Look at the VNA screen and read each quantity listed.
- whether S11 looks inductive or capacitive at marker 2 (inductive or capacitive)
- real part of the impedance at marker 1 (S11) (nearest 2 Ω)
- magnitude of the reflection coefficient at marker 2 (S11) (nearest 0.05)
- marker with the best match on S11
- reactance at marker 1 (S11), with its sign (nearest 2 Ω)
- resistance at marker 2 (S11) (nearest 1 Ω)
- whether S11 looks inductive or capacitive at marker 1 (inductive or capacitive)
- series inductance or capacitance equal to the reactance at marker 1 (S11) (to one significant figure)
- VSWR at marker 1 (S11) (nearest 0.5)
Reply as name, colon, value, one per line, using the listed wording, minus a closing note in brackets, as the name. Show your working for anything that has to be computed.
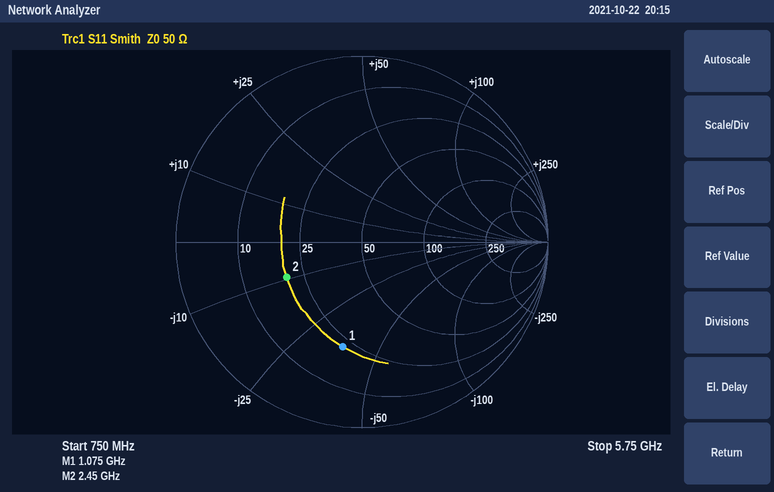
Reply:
whether S11 looks inductive or capacitive at marker 2: capacitive
real part of the impedance at marker 1 (S11): 22 Ω
magnitude of the reflection coefficient at marker 2 (S11): 0.45
marker with the best match on S11: marker 2
reactance at marker 1 (S11), with its sign: -36 Ω
resistance at marker 2 (S11): 20 Ω
whether S11 looks inductive or capacitive at marker 1: capacitive
series inductance or capacitance equal to the reactance at marker 1 (S11): C = 1/(2π × 1.075 GHz × 36 Ω) ≈ 4 pF
VSWR at marker 1 (S11): 3.5
